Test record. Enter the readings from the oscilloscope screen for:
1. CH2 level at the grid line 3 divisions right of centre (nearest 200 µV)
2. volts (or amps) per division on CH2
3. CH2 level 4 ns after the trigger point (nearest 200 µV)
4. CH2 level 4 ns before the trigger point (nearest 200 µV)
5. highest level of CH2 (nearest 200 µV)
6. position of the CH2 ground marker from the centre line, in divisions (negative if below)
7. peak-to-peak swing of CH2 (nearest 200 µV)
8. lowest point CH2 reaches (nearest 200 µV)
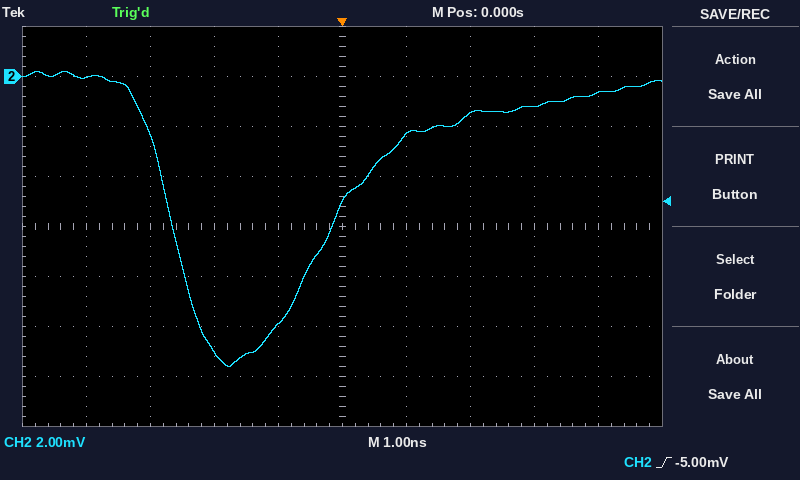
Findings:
-1.2 mV
2 mV
-600 µV
0.0 mV
200 µV
+3.0 div
11.8 mV
-11.6 mV
